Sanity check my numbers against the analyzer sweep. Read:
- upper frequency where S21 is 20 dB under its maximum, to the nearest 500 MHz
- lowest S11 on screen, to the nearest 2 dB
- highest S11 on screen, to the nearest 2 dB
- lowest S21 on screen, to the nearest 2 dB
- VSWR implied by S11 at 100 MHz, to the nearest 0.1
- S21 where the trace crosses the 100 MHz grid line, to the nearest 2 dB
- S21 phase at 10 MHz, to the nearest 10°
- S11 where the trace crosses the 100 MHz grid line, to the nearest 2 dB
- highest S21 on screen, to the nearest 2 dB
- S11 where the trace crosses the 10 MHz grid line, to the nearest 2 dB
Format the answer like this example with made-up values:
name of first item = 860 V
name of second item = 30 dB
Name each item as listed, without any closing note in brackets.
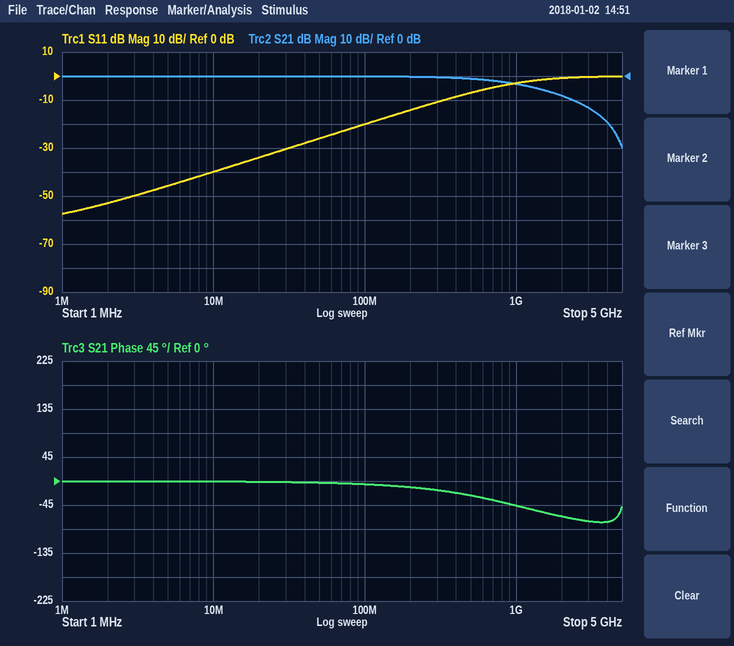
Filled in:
upper frequency where S21 is 20 dB under its maximum, to the nearest 500 MHz = 4.0 GHz
lowest S11 on screen, to the nearest 2 dB = -58 dB
highest S11 on screen, to the nearest 2 dB = 0 dB
lowest S21 on screen, to the nearest 2 dB = -30 dB
VSWR implied by S11 at 100 MHz, to the nearest 0.1 = 1.2
S21 where the trace crosses the 100 MHz grid line, to the nearest 2 dB = 0 dB
S21 phase at 10 MHz, to the nearest 10° = 0°
S11 where the trace crosses the 100 MHz grid line, to the nearest 2 dB = -20 dB
highest S21 on screen, to the nearest 2 dB = 0 dB
S11 where the trace crosses the 10 MHz grid line, to the nearest 2 dB = -40 dB
